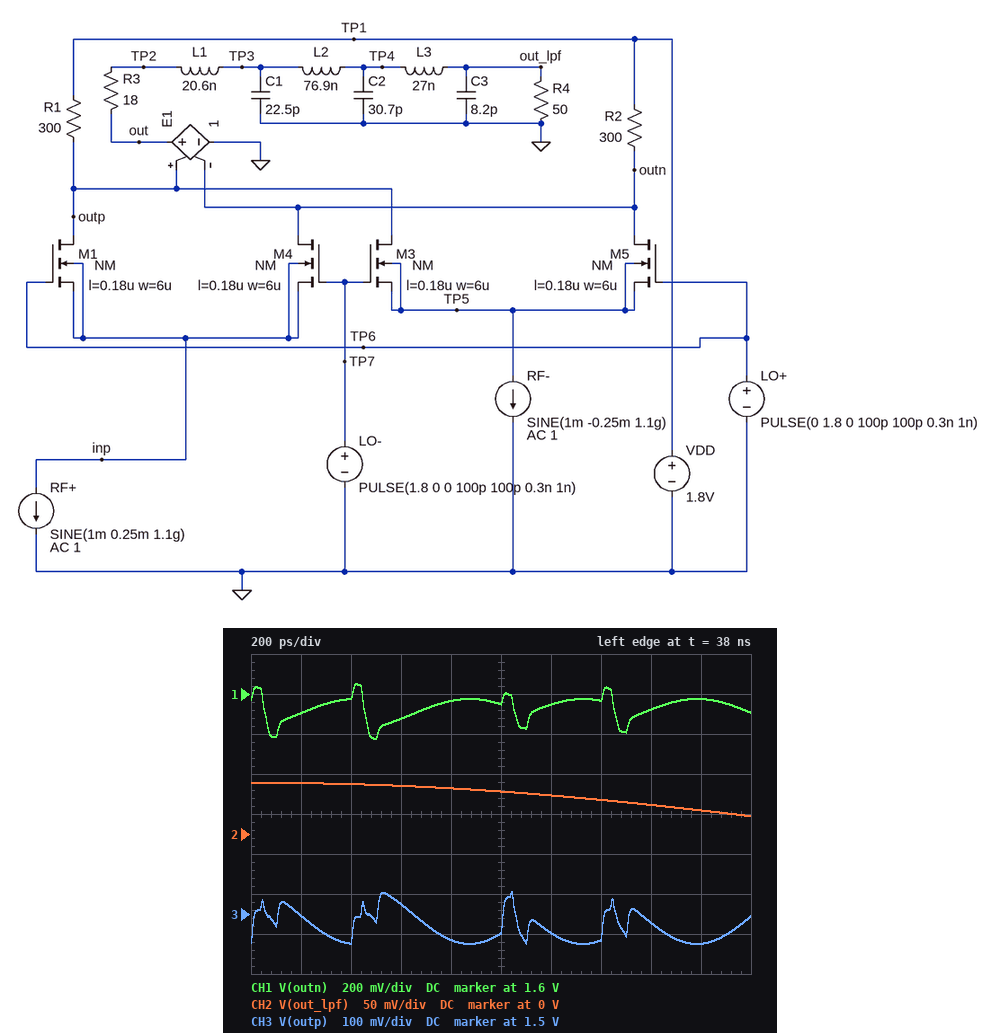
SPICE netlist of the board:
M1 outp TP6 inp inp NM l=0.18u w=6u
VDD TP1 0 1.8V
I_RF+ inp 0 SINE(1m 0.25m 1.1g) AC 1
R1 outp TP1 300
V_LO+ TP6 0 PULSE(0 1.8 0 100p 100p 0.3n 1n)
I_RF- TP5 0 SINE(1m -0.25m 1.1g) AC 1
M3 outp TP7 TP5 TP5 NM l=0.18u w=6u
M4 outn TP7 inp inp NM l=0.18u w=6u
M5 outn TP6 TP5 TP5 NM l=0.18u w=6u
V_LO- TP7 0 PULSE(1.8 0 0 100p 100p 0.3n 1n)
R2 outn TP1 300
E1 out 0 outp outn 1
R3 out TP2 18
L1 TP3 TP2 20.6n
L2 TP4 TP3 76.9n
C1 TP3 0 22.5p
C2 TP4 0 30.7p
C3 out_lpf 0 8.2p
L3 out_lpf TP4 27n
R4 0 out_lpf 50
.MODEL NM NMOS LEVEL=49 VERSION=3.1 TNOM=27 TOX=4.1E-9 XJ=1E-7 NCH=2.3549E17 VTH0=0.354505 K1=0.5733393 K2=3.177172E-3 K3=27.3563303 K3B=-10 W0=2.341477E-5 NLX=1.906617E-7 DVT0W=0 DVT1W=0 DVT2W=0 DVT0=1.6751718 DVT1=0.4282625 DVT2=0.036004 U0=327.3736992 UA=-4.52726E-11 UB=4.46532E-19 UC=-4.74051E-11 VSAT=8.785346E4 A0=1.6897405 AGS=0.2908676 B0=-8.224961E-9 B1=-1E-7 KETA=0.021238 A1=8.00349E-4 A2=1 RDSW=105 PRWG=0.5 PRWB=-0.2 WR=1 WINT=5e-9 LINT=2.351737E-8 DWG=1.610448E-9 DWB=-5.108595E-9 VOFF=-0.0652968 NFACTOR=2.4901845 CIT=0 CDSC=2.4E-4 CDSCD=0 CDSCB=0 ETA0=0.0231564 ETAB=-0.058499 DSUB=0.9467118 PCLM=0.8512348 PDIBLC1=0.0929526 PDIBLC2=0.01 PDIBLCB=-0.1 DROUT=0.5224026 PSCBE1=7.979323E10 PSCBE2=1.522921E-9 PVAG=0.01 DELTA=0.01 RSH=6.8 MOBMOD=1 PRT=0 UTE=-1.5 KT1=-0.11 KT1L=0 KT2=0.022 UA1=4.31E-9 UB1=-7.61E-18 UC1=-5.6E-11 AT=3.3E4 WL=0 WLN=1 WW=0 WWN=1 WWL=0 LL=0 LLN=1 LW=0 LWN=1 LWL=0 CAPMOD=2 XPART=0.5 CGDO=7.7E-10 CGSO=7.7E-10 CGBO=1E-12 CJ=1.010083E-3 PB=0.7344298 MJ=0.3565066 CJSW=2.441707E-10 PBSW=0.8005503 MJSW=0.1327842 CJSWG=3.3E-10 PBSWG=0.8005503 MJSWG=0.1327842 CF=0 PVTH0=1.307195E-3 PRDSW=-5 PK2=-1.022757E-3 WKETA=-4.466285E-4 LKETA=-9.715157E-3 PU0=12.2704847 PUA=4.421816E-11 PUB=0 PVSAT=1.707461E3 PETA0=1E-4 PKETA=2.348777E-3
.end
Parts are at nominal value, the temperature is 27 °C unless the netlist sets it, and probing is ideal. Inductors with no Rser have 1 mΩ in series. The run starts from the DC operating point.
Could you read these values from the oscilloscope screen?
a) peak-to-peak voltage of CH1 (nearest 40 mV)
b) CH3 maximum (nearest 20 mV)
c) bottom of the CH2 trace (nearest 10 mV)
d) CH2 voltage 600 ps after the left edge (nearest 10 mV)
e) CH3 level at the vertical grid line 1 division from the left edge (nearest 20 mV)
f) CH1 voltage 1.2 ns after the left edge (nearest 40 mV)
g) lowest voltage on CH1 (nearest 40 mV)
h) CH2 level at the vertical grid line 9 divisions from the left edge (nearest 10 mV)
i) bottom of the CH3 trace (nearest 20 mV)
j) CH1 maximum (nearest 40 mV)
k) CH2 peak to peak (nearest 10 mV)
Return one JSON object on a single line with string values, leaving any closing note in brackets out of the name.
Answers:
{"peak-to-peak voltage of CH1": "280 mV", "CH3 maximum": "1.56 V", "bottom of the CH2 trace": "20 mV", "CH2 voltage 600 ps after the left edge": "60 mV", "CH3 level at the vertical grid line 1 division from the left edge": "1.50 V", "CH1 voltage 1.2 ns after the left edge": "1.56 V", "lowest voltage on CH1": "1.36 V", "CH2 level at the vertical grid line 9 divisions from the left edge": "30 mV", "bottom of the CH3 trace": "1.42 V", "CH1 maximum": "1.64 V", "CH2 peak to peak": "40 mV"}
